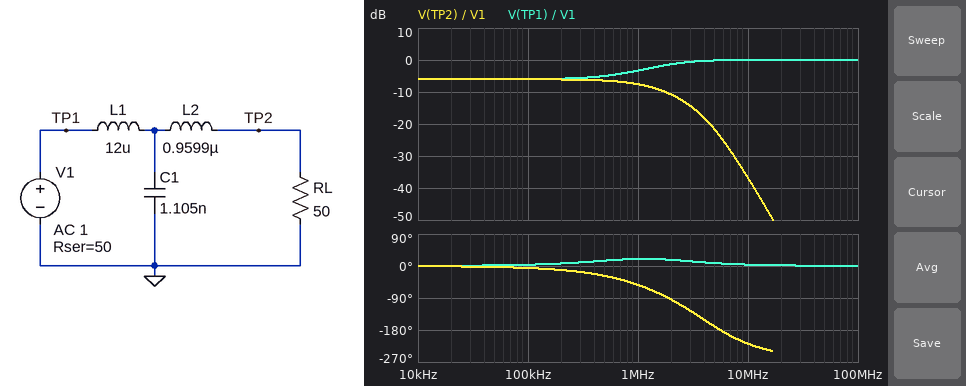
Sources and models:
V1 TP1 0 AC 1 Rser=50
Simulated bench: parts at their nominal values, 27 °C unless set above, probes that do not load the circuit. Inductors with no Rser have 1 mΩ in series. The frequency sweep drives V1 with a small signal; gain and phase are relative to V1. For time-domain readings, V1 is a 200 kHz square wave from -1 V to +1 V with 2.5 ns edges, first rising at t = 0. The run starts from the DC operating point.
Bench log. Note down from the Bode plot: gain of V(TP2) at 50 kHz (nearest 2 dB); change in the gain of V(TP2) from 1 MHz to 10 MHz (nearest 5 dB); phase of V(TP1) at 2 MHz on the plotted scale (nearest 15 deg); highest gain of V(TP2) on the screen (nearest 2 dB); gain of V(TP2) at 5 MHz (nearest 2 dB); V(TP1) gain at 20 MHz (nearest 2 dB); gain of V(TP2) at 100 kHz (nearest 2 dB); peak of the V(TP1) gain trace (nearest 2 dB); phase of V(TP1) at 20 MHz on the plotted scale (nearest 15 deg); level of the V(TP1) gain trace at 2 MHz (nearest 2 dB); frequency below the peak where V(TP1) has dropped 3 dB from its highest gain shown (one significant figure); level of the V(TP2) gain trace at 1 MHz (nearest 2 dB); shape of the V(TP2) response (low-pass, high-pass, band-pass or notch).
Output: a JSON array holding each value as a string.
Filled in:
["-6 dB", "-30 dB", "15 deg", "-6 dB", "-22 dB", "0 dB", "-6 dB", "0 dB", "0 deg", "-2 dB", "1 MHz", "-8 dB", "low-pass"]
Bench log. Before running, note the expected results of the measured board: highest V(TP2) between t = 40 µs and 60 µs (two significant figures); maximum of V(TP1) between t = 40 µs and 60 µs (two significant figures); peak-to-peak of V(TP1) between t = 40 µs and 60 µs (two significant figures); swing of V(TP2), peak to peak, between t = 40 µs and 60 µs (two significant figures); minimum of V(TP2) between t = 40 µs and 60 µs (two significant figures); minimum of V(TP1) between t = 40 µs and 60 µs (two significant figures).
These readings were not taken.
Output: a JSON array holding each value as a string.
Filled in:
["500 mV", "1.5 V", "3.0 V", "1.0 V", "-500 mV", "-1.5 V"]
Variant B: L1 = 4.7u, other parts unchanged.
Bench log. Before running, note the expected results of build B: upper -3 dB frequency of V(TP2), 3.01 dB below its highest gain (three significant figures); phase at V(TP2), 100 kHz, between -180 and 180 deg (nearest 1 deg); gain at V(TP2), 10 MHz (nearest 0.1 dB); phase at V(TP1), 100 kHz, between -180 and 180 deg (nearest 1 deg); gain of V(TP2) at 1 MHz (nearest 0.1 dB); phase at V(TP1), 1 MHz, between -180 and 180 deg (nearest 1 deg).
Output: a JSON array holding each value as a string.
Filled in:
["3.49 MHz", "-3 deg", "-28.5 dB", "1 deg", "-6.2 dB", "10 deg"]
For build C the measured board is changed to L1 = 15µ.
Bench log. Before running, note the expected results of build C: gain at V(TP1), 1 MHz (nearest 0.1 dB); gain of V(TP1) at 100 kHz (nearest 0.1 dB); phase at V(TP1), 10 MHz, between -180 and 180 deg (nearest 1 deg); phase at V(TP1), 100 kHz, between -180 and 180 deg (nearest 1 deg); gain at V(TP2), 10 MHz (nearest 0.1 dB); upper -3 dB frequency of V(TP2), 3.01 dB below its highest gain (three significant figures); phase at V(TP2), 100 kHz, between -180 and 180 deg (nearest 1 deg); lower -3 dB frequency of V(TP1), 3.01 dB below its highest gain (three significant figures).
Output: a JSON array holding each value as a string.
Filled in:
["-2.5 dB", "-5.9 dB", "3 deg", "5 deg", "-38.8 dB", "1.17 MHz", "-7 deg", "851 kHz"]
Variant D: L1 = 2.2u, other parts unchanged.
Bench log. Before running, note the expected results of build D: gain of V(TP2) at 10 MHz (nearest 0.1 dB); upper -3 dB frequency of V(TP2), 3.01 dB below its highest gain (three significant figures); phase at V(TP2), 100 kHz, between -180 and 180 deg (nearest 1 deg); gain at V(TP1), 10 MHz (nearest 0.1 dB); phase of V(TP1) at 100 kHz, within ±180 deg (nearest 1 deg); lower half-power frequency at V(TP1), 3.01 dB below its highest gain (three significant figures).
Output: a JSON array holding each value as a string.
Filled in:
["-21.9 dB", "5.20 MHz", "-2 deg", "-0.7 dB", "0 deg", "6.13 MHz"]
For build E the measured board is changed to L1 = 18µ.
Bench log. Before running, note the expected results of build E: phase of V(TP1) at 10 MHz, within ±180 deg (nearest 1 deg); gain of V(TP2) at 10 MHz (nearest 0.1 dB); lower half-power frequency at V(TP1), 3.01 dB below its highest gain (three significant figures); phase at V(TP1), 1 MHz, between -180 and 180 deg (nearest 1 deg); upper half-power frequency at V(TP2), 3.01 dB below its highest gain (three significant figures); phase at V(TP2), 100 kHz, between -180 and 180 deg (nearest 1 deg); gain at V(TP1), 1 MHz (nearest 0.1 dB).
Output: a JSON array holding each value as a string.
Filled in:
["3 deg", "-40.4 dB", "694 kHz", "19 deg", "964 kHz", "-8 deg", "-2.0 dB"]
